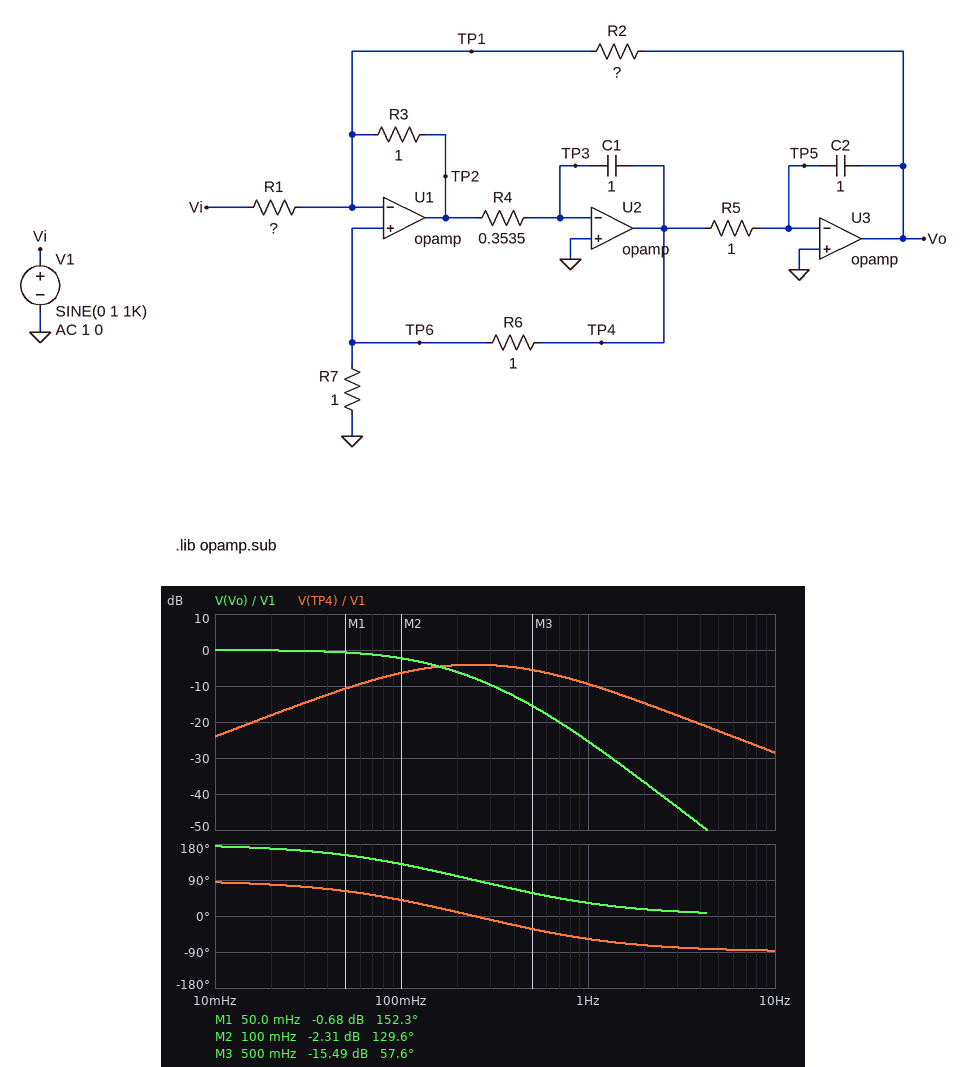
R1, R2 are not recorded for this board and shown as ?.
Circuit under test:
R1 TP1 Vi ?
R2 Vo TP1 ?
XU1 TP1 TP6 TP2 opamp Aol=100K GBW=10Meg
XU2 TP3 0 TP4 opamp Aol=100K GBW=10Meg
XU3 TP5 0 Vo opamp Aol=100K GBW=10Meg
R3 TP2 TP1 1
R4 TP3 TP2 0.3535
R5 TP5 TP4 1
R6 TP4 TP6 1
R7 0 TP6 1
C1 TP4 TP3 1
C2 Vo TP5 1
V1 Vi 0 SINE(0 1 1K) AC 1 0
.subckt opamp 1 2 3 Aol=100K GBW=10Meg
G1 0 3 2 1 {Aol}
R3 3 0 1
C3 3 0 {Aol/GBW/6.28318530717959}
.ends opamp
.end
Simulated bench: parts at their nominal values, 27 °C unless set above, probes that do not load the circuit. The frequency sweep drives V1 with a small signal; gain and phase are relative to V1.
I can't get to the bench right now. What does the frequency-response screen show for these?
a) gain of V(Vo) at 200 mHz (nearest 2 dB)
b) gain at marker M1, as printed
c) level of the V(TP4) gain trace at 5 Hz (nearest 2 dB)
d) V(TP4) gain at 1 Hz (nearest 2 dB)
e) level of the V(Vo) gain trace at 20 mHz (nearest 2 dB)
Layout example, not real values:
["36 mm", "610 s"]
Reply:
["-6 dB", "-0.68 dB", "-22 dB", "-10 dB", "0 dB"]
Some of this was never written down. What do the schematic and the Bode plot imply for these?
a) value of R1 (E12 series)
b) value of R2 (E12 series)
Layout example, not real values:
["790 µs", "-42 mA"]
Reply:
["1.2 Ω", "1.2 Ω"]
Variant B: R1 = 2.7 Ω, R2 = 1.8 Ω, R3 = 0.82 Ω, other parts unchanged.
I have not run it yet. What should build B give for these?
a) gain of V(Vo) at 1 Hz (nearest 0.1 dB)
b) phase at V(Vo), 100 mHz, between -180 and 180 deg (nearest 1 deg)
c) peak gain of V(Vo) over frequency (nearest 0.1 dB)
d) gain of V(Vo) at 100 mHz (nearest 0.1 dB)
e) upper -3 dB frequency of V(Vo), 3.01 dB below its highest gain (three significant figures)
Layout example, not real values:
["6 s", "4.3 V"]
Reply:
["-33.6 dB", "120 deg", "-3.5 dB", "-6.4 dB", "102 mHz"]
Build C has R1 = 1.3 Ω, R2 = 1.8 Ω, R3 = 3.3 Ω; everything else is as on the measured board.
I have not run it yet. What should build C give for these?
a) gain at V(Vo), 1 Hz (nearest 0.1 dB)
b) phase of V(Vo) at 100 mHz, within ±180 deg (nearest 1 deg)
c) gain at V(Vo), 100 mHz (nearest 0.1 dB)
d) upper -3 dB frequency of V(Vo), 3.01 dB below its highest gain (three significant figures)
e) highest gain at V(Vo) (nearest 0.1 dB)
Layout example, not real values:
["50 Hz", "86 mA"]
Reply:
["-18.3 dB", "135 deg", "0.5 dB", "119 mHz", "2.8 dB"]
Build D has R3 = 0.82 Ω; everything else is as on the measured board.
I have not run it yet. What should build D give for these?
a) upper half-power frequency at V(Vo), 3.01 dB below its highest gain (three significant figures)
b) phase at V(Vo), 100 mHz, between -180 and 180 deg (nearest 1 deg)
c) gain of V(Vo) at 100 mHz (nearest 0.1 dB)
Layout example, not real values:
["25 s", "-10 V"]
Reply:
["110 mHz", "126 deg", "-2.6 dB"]
